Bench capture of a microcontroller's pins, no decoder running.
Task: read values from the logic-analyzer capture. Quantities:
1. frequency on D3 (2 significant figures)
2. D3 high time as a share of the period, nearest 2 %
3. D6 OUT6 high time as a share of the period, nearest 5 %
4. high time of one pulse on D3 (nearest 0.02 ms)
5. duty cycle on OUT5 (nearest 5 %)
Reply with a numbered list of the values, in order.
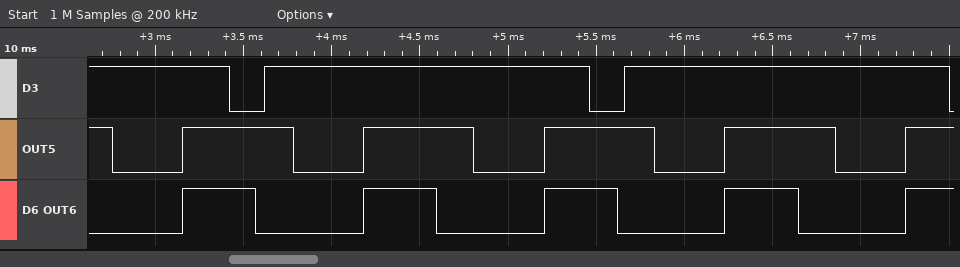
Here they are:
1. 490 Hz
2. 90 %
3. 40 %
4. 1.84 ms
5. 60 %
